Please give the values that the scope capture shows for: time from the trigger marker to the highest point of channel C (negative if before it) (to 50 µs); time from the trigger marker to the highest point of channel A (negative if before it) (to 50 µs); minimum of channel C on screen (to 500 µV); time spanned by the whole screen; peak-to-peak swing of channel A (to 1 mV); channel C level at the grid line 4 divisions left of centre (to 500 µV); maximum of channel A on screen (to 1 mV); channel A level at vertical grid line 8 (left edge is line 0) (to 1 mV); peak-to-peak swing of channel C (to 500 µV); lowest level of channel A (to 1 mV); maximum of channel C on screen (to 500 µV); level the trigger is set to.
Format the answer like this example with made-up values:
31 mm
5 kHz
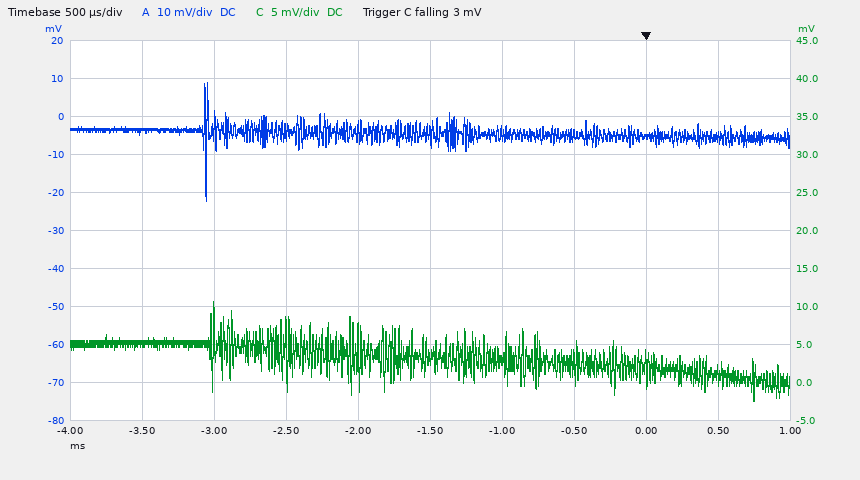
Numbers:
-3.00 ms
-3.05 ms
-2.5 mV
5 ms
31 mV
5.0 mV
9 mV
-5 mV
13.0 mV
-22 mV
10.5 mV
3 mV
